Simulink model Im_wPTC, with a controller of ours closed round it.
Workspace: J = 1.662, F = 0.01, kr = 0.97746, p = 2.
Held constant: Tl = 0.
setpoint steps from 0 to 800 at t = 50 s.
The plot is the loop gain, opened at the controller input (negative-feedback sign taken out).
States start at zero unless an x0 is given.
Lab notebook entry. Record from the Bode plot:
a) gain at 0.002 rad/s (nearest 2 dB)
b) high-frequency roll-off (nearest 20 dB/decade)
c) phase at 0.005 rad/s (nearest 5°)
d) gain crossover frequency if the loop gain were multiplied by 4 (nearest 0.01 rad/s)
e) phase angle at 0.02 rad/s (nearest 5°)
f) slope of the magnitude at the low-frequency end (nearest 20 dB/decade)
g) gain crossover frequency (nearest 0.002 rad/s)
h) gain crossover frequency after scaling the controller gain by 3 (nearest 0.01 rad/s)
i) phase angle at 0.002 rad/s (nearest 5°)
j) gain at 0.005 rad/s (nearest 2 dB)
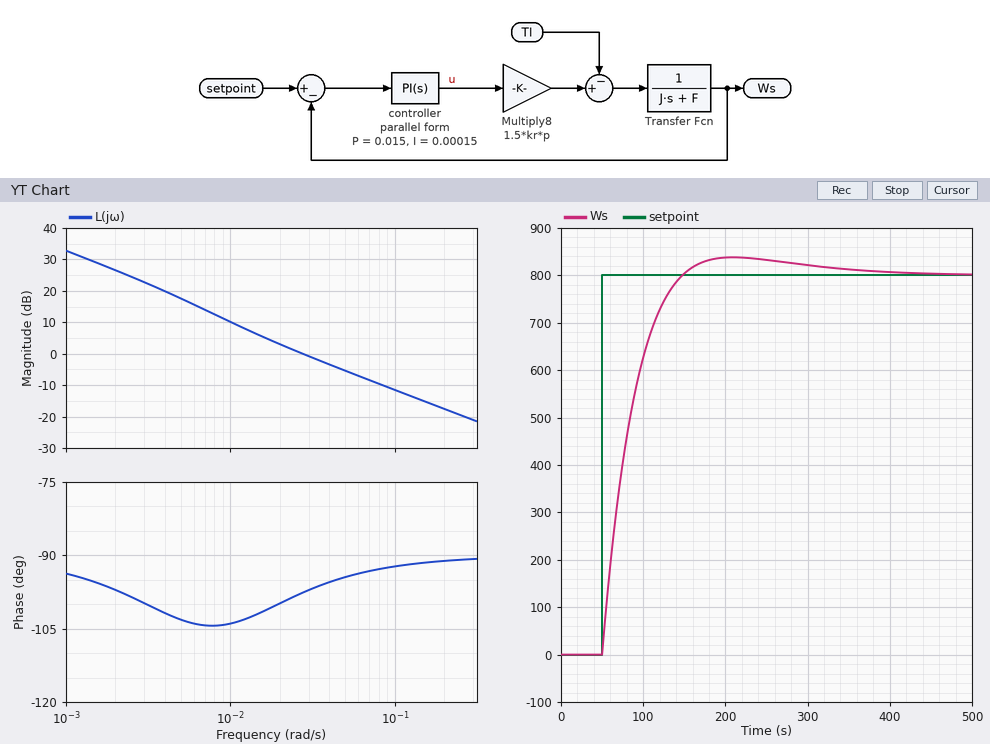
26 dB
-20 dB/decade
-105°
0.11 rad/s
-100°
-20 dB/decade
0.028 rad/s
0.08 rad/s
-95°
18 dB
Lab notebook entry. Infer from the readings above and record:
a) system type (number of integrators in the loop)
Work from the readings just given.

1
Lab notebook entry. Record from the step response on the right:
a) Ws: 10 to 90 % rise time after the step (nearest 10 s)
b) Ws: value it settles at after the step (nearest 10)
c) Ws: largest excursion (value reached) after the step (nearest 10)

60 s
800
840
